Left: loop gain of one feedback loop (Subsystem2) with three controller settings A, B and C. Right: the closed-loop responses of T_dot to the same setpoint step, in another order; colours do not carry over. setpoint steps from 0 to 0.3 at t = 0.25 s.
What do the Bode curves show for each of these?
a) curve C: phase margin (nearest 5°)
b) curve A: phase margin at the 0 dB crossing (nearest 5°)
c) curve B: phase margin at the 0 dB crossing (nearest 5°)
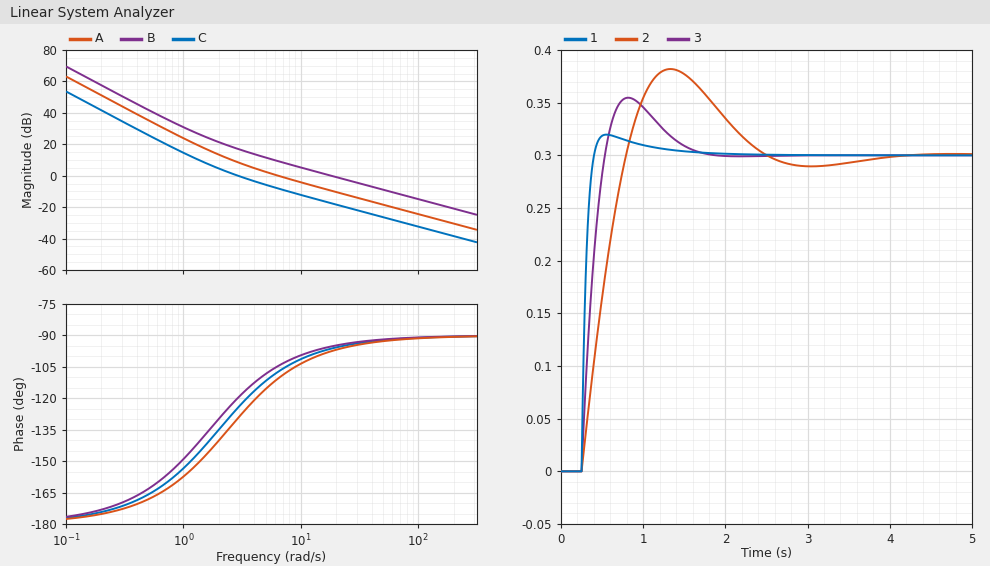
55°
70°
85°
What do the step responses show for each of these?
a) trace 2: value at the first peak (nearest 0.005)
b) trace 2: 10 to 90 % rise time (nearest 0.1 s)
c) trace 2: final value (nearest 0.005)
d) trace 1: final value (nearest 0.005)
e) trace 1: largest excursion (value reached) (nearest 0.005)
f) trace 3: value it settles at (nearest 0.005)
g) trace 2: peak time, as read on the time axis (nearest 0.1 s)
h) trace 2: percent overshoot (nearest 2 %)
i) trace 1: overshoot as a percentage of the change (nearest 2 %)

0.380
0.4 s
0.300
0.300
0.320
0.300
1.3 s
28 %
6 %
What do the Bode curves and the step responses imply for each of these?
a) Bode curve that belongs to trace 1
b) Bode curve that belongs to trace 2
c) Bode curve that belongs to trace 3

B
C
A
